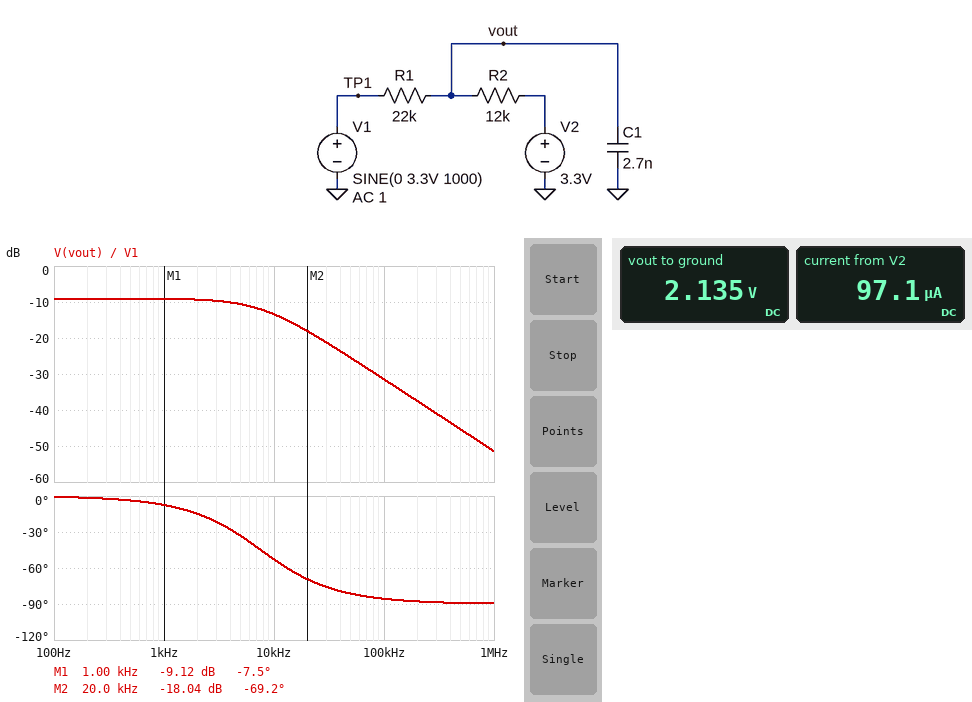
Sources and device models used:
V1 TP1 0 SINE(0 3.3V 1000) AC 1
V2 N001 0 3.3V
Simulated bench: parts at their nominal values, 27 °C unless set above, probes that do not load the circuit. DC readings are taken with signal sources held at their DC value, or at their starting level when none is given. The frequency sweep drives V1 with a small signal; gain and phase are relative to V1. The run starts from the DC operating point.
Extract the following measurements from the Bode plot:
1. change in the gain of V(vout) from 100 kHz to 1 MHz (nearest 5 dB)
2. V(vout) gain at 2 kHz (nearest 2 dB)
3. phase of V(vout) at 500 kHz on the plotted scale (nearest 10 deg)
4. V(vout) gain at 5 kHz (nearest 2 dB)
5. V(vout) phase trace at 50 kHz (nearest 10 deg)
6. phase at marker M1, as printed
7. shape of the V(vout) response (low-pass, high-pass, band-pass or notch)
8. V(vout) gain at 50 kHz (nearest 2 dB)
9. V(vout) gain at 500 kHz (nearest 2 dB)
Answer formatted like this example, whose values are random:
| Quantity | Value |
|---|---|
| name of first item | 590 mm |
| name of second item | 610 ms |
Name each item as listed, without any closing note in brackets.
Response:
| Quantity | Value |
|---|---|
| change in the gain of V(vout) from 100 kHz to 1 MHz | -20 dB |
| V(vout) gain at 2 kHz | -10 dB |
| phase of V(vout) at 500 kHz on the plotted scale | -90 deg |
| V(vout) gain at 5 kHz | -10 dB |
| V(vout) phase trace at 50 kHz | -80 deg |
| phase at marker M1, as printed | -7.5 deg |
| shape of the V(vout) response | low-pass |
| V(vout) gain at 50 kHz | -26 dB |
| V(vout) gain at 500 kHz | -46 dB |
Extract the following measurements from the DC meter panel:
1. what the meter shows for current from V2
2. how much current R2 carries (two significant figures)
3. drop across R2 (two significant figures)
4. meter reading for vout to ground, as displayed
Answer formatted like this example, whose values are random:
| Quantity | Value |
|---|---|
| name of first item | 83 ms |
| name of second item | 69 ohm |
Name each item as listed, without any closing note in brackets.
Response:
| Quantity | Value |
|---|---|
| what the meter shows for current from V2 | 97.1 µA |
| how much current R2 carries | 97 µA |
| drop across R2 | 1.2 V |
| meter reading for vout to ground, as displayed | 2.135 V |
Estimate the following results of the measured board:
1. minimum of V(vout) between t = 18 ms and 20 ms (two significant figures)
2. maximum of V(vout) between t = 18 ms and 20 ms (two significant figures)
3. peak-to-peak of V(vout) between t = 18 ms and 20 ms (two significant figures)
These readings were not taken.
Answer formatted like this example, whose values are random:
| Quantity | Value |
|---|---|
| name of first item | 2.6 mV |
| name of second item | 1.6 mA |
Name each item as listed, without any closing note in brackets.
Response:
| Quantity | Value |
|---|---|
| minimum of V(vout) between t = 18 ms and 20 ms | 980 mV |
| maximum of V(vout) between t = 18 ms and 20 ms | 3.3 V |
| peak-to-peak of V(vout) between t = 18 ms and 20 ms | 2.3 V |
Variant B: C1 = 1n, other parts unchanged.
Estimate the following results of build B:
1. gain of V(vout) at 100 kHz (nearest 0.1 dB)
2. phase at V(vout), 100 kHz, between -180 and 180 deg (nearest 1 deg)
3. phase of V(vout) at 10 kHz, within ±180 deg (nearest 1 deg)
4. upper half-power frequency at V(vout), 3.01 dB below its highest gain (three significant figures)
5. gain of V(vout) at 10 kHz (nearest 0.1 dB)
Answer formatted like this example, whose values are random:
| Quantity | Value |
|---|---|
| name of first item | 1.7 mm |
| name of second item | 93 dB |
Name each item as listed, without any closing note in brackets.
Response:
| Quantity | Value |
|---|---|
| gain of V(vout) at 100 kHz | -23.0 dB |
| phase at V(vout), 100 kHz, between -180 and 180 deg | -78 deg |
| phase of V(vout) at 10 kHz, within ±180 deg | -26 deg |
| upper half-power frequency at V(vout), 3.01 dB below its highest gain | 20.5 kHz |
| gain of V(vout) at 10 kHz | -10.0 dB |
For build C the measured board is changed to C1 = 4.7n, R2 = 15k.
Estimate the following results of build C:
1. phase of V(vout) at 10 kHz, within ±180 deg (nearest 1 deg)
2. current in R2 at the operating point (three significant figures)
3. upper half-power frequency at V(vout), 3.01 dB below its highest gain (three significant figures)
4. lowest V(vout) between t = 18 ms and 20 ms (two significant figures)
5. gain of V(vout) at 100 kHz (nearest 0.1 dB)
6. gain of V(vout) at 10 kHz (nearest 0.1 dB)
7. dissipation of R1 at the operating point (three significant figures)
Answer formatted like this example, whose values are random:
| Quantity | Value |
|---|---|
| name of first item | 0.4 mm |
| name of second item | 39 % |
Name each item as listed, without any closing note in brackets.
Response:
| Quantity | Value |
|---|---|
| phase of V(vout) at 10 kHz, within ±180 deg | -69 deg |
| current in R2 at the operating point | 89.2 µA |
| upper half-power frequency at V(vout), 3.01 dB below its highest gain | 3.80 kHz |
| lowest V(vout) between t = 18 ms and 20 ms | 670 mV |
| gain of V(vout) at 100 kHz | -36.3 dB |
| gain of V(vout) at 10 kHz | -16.8 dB |
| dissipation of R1 at the operating point | 175 µW |
